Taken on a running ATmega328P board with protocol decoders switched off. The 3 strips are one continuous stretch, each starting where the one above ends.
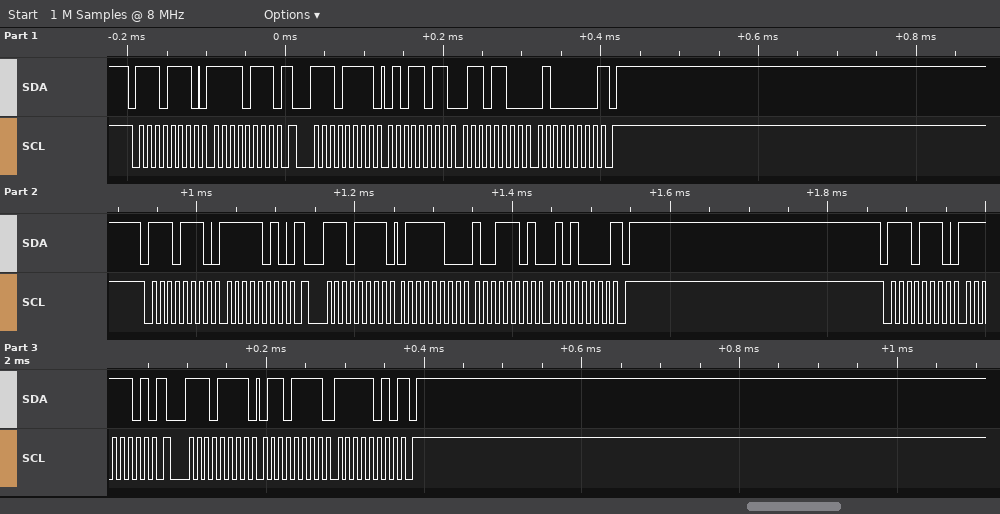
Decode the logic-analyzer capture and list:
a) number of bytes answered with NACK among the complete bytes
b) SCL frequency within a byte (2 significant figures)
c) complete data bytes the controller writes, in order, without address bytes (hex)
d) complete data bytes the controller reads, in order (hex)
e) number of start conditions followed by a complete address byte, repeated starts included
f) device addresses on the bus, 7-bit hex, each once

3
100 kHz
F7 FA FD
5B 6C 40 7C 9D 50 6F FA
6
0x77
